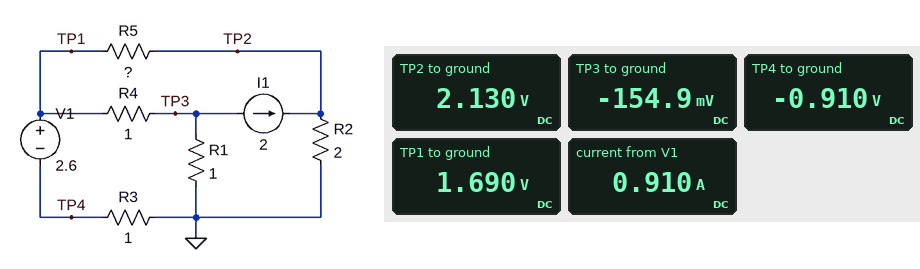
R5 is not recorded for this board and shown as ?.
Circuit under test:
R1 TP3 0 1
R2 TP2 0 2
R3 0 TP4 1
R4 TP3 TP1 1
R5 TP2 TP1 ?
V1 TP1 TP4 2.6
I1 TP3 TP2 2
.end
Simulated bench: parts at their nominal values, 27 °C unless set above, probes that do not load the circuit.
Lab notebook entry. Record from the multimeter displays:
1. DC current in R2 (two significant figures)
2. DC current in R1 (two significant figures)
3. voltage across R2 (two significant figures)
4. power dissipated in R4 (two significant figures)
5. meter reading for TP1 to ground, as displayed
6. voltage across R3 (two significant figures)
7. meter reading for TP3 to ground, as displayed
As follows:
1.1 A
150 mA
2.1 V
3.4 W
1.690 V
910 mV
-154.9 mV
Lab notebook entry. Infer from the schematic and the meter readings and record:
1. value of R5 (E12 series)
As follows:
0.47 Ω
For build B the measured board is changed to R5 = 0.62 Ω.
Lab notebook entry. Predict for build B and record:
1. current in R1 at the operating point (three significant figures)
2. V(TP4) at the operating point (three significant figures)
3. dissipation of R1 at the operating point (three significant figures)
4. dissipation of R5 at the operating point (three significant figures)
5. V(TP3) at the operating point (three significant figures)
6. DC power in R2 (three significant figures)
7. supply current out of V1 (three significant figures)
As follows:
169 mA
-938 mV
28.6 mW
494 mW
-169 mV
2.45 W
938 mA
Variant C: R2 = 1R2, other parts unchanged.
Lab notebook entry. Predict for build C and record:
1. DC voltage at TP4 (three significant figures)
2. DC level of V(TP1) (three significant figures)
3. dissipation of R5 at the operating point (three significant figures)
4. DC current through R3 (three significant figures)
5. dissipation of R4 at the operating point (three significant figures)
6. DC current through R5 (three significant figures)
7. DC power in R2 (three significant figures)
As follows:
-1.15 V
1.45 V
153 mW
1.15 A
2.97 W
571 mA
2.45 W
